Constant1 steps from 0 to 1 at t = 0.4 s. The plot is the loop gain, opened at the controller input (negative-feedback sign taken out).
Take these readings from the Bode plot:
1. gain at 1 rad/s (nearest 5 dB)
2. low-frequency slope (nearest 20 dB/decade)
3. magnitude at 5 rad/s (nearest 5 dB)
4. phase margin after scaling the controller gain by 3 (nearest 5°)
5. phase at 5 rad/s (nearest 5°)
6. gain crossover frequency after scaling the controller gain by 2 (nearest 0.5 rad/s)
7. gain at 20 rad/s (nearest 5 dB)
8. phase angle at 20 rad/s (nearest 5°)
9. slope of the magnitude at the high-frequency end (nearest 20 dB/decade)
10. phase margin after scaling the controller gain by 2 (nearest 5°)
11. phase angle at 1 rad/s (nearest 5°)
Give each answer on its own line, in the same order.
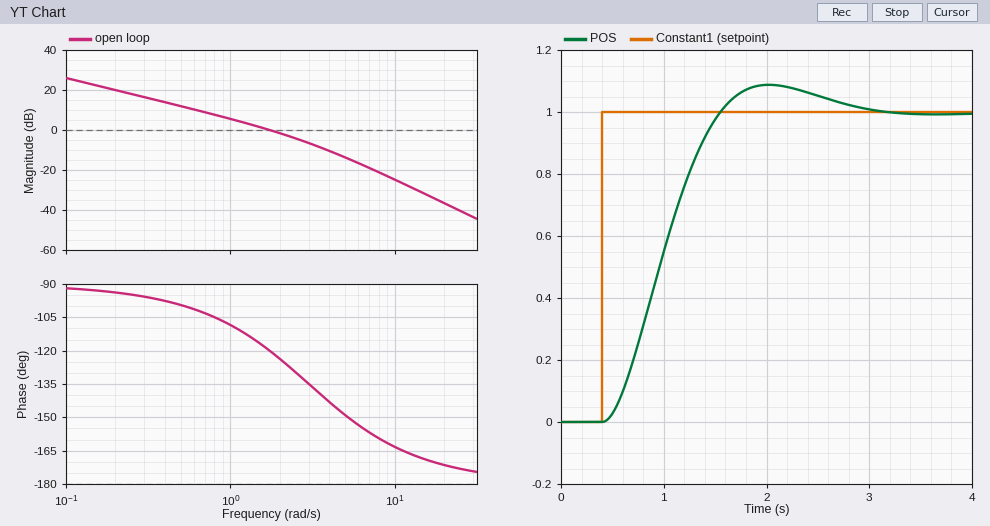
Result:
5 dB
-20 dB/decade
-15 dB
40°
-150°
3.0 rad/s
-35 dB
-170°
-40 dB/decade
45°
-110°
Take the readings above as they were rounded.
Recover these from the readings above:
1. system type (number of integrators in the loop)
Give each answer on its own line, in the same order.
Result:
1
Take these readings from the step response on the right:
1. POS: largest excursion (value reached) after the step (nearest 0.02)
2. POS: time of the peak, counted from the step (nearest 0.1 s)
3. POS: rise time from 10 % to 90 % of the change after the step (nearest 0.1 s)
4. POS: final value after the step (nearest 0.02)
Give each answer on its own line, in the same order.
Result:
1.08
1.6 s
0.8 s
1.00
